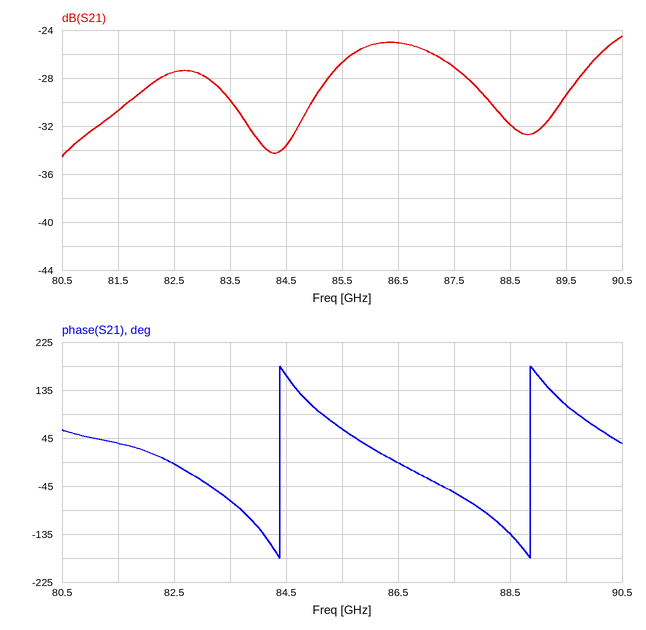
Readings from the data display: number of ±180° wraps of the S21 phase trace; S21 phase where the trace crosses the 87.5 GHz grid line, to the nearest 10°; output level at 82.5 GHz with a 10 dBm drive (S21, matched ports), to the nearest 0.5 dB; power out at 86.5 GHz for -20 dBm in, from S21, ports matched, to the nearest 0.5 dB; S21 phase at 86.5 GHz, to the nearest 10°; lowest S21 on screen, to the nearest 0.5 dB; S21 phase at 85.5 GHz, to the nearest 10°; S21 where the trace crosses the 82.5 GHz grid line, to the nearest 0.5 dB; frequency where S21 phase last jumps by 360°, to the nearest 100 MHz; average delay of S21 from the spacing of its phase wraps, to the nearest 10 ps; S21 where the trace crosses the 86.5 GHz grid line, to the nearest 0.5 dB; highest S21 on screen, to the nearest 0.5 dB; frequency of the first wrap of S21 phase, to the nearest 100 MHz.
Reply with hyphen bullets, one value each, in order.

- 2
- -60°
- -17.5 dBm
- -45.0 dBm
- 0°
- -34.5 dB
- 60°
- -27.5 dB
- 88.9 GHz
- 220 ps
- -25.0 dB
- -24.5 dB
- 84.4 GHz
